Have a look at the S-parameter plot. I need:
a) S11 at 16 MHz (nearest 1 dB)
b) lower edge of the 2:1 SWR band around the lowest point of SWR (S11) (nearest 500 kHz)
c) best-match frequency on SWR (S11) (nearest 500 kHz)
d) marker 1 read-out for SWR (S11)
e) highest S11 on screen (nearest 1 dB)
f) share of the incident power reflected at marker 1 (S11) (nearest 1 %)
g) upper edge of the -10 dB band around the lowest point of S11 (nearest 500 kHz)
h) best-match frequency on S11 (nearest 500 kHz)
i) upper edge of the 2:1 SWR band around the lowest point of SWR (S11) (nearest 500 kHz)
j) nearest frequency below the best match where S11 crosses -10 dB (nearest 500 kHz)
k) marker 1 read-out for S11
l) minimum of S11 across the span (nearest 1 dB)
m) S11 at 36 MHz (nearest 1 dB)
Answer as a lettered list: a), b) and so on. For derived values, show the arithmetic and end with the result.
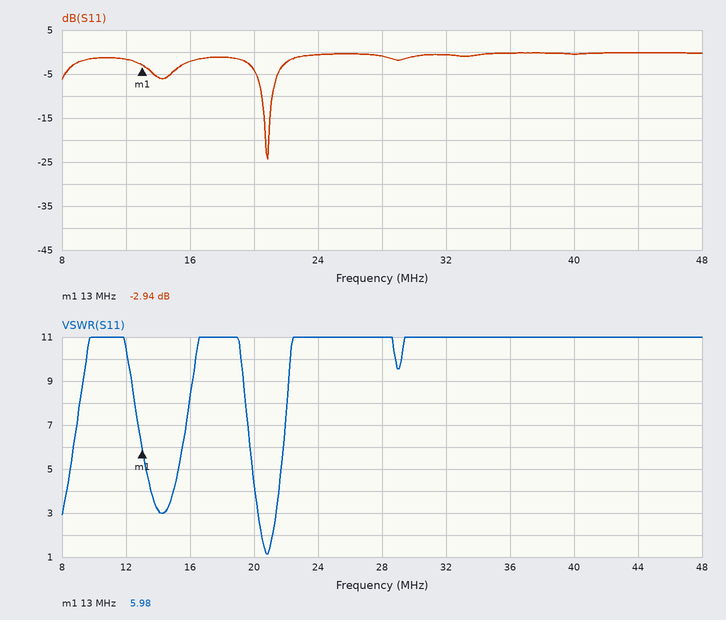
a) -2 dB
b) 20.5 MHz
c) 21.0 MHz
d) 5.98
e) 0 dB
f) 10^(-2.94/10) ≈ 51 %
g) 21.0 MHz
h) 21.0 MHz
i) 21.0 MHz
j) 20.5 MHz
k) -2.94 dB
l) -24 dB
m) 0 dB
